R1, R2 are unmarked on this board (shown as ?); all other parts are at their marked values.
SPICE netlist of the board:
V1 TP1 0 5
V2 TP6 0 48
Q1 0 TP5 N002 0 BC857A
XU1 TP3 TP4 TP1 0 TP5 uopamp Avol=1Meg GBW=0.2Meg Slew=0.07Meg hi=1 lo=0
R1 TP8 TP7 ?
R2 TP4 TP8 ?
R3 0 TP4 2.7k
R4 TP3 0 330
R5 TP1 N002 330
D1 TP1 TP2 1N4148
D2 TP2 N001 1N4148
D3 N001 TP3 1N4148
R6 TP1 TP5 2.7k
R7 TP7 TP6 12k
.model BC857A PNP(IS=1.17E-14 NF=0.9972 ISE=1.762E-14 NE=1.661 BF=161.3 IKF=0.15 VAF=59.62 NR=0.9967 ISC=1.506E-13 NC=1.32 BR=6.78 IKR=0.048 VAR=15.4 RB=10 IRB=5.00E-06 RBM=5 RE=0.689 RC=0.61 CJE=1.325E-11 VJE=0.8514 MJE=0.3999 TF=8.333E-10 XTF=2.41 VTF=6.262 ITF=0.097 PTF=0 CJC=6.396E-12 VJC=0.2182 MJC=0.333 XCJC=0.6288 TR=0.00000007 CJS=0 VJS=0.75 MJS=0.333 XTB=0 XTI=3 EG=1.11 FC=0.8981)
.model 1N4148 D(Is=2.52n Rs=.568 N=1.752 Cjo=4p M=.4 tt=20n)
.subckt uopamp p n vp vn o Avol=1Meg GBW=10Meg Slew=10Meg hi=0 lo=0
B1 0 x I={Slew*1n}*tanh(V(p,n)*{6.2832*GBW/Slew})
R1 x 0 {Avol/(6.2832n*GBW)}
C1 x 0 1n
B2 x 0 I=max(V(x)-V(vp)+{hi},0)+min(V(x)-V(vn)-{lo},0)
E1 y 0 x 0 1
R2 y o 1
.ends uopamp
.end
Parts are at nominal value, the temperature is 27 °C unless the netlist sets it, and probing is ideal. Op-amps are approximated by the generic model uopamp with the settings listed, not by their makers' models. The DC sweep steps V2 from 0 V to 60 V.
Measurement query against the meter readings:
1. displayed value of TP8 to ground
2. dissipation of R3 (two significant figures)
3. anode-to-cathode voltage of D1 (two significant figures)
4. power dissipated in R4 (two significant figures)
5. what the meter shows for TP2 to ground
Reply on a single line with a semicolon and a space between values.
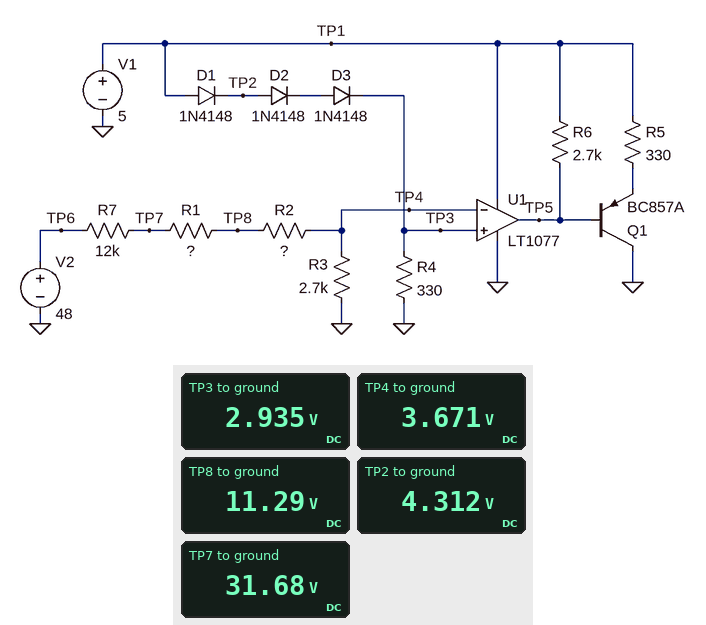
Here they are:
11.29 V; 5.0 mW; 690 mV; 26 mW; 4.312 V
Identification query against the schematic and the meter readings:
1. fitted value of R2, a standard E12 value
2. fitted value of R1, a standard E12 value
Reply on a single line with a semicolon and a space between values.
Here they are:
5.6 kΩ; 15 kΩ
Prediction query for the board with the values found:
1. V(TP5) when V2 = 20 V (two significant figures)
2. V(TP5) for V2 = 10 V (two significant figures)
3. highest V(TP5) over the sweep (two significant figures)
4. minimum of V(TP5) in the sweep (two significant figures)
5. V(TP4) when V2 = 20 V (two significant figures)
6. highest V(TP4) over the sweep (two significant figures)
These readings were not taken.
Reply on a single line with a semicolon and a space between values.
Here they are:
4.0 V; 4.0 V; 4.0 V; 1.9 mV; 1.5 V; 4.6 V
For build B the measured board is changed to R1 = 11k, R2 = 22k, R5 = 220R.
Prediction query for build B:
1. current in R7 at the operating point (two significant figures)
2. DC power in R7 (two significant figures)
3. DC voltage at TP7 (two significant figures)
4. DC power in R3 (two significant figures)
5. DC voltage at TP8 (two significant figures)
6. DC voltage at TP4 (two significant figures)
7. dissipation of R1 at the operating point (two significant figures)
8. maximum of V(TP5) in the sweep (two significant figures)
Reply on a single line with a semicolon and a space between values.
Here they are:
1.0 mA; 12 mW; 36 V; 2.7 mW; 25 V; 2.7 V; 11 mW; 4.0 V
